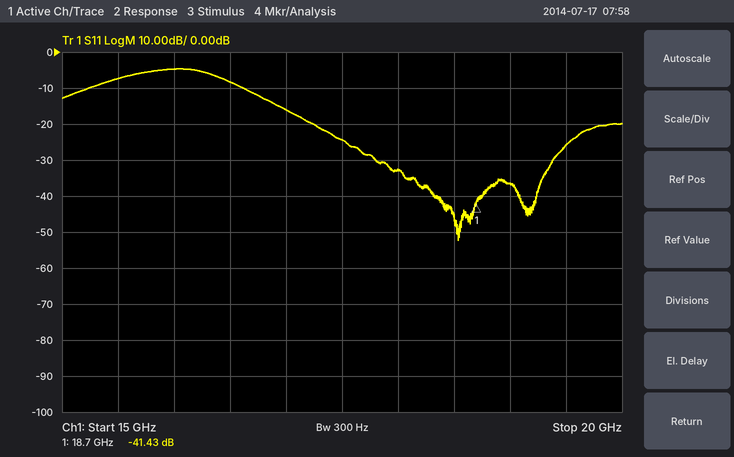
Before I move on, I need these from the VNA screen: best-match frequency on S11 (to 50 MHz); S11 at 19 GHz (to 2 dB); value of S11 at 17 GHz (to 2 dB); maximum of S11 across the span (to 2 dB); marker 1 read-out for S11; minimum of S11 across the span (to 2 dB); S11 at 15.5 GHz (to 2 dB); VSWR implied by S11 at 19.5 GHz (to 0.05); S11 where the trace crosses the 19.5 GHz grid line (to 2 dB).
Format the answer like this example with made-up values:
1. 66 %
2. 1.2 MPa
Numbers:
1. 18.55 GHz
2. -36 dB
3. -16 dB
4. -4 dB
5. -41.43 dB
6. -52 dB
7. -8 dB
8. 1.10
9. -26 dB
